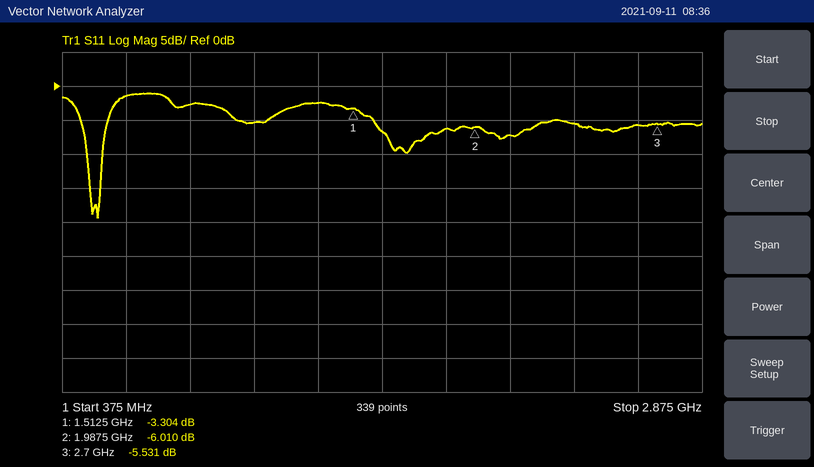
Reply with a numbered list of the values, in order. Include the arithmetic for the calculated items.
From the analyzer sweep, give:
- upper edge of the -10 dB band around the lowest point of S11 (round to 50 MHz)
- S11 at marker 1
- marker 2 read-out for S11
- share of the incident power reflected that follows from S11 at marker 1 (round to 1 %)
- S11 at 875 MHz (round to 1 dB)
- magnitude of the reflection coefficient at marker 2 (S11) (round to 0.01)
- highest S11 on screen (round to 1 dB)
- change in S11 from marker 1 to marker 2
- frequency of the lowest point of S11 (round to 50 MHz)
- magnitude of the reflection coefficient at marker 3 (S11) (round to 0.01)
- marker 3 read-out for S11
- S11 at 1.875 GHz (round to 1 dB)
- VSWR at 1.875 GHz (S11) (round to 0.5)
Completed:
1. 550 MHz
2. -3.304 dB
3. -6.010 dB
4. 10^(-3.304/10) ≈ 47 %
5. -3 dB
6. 10^(-6.01/20) ≈ 0.50
7. -1 dB
8. -6.01 − (-3.304) = -2.706 dB
9. 500 MHz
10. 10^(-5.531/20) ≈ 0.53
11. -5.531 dB
12. -6 dB
13. |Γ| = 10^(-6/20) = 0.5012; VSWR = (1 + 0.5012)/(1 − 0.5012) ≈ 3.0
